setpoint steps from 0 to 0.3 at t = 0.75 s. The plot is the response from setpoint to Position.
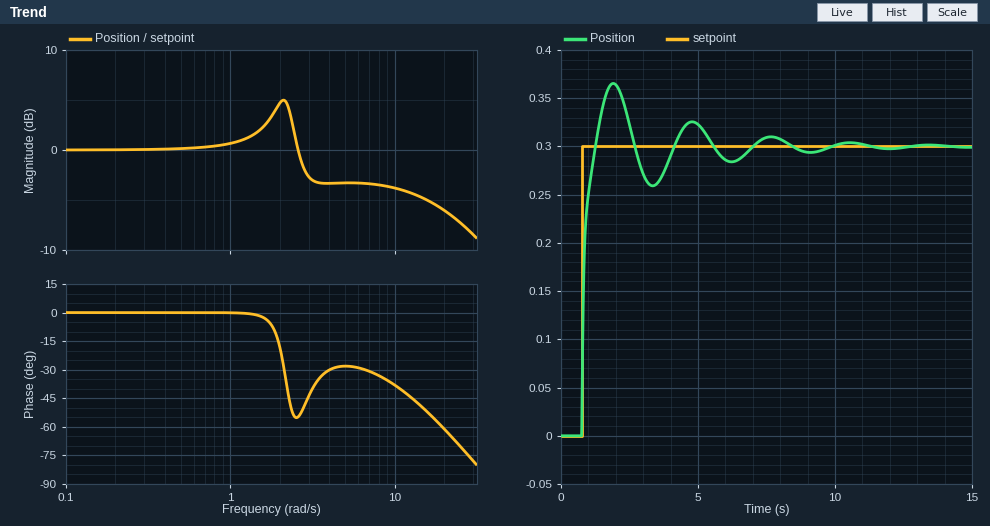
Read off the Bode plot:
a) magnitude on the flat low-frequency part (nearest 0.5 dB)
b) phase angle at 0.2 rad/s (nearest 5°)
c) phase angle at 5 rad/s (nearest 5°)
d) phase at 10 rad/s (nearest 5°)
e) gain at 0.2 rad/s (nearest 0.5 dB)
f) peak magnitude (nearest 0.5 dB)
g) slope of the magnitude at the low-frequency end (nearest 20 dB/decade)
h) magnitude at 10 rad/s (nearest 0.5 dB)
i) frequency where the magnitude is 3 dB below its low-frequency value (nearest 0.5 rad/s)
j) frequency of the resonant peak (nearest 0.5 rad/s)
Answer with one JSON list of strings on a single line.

["0.0 dB", "0°", "-30°", "-40°", "0.0 dB", "5.0 dB", "0 dB/decade", "-4.0 dB", "3.0 rad/s", "2.0 rad/s"]
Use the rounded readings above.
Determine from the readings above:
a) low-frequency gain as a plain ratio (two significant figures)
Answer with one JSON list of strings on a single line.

["1.0"]
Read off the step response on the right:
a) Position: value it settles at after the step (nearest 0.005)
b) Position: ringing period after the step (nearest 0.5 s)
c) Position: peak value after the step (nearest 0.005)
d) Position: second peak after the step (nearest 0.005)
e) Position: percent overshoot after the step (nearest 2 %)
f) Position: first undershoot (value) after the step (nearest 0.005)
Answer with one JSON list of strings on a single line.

["0.300", "3.0 s", "0.365", "0.325", "22 %", "0.260"]
